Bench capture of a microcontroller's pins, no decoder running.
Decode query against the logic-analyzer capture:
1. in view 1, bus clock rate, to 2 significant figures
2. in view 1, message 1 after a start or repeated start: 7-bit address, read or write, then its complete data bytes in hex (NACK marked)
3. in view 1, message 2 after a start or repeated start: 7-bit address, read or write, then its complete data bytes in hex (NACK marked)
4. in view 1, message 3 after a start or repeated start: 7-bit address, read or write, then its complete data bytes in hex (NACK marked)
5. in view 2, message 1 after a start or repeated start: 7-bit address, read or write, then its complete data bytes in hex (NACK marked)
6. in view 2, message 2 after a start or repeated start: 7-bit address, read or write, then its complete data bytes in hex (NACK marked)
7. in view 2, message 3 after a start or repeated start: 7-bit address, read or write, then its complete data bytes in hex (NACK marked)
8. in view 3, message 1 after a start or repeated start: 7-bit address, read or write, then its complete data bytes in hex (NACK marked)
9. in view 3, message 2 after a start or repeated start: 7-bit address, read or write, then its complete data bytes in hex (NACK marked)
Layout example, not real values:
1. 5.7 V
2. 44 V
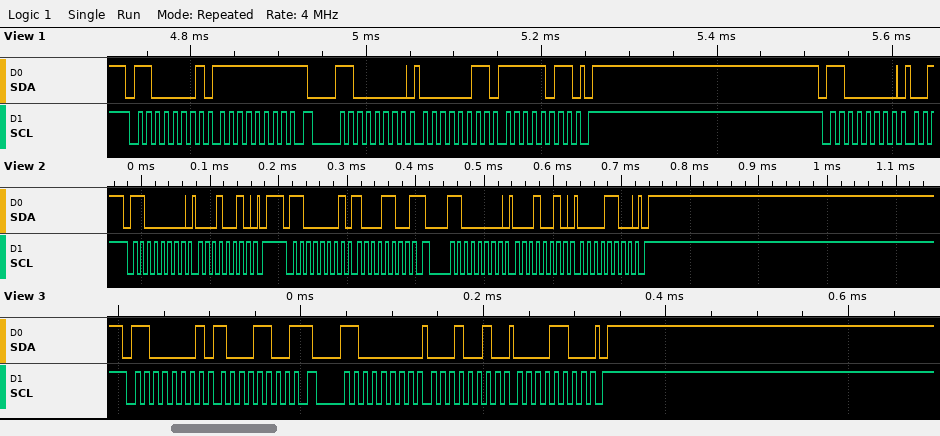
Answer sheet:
1. 100 kHz
2. 0x60 read: FF NACK
3. 0x60 write: 03 FB
4. 0x60 write
5. 0x60 write: 12
6. 0x60 read: 8C NACK
7. 0x60 write: 12 0C
8. 0x60 read: 8C NACK
9. 0x60 write: 12 0C
